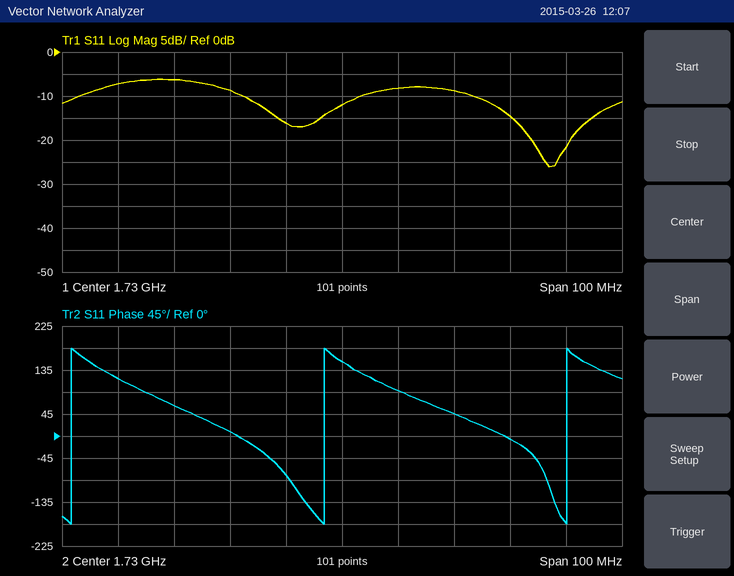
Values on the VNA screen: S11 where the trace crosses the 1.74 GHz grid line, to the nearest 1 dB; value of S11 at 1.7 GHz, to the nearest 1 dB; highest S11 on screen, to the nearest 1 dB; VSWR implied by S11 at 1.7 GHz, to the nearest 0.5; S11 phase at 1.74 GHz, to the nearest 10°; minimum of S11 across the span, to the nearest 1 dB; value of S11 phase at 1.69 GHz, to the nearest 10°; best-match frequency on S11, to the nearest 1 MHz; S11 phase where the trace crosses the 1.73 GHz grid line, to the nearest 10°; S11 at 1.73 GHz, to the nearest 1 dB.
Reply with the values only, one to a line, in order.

-8 dB
-6 dB
-6 dB
3.0
90°
-26 dB
120°
1.767 GHz
150°
-12 dB
